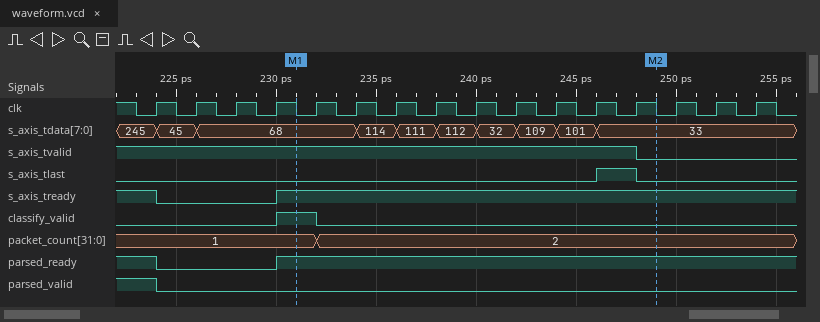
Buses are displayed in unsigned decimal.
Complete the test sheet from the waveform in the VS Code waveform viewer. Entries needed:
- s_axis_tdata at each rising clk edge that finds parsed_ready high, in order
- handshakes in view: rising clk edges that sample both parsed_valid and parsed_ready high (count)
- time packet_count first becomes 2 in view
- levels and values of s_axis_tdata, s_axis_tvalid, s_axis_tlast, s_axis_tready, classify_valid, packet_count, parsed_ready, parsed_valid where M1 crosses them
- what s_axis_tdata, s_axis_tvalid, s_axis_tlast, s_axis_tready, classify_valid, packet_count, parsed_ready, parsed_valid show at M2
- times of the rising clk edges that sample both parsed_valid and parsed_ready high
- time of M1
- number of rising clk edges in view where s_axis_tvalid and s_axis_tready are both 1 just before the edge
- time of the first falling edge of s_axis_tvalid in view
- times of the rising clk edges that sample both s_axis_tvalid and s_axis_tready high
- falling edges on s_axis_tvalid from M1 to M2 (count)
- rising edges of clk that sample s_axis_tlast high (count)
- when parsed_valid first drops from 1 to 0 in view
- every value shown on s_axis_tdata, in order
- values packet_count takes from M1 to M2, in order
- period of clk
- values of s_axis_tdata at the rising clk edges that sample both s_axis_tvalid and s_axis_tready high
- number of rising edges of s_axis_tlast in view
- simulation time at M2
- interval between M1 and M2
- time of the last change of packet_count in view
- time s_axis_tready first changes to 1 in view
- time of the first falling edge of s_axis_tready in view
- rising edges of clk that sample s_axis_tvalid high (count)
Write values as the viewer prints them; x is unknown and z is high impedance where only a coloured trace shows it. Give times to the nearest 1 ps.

245, 68, 68, 114, 111, 112, 32, 109, 101, 33, 33, 33, 33
1
232 ps
s_axis_tdata=68, s_axis_tvalid=1, s_axis_tlast=0, s_axis_tready=1, classify_valid=1, packet_count=1, parsed_ready=1, parsed_valid=0
s_axis_tdata=33, s_axis_tvalid=0, s_axis_tlast=0, s_axis_tready=1, classify_valid=0, packet_count=2, parsed_ready=1, parsed_valid=0
224 ps
231 ps
10
248 ps
224 ps, 232 ps, 234 ps, 236 ps, 238 ps, 240 ps, 242 ps, 244 ps, 246 ps, 248 ps
1
1
224 ps
245, 45, 68, 114, 111, 112, 32, 109, 101, 33
1, 2
2 ps
245, 68, 68, 114, 111, 112, 32, 109, 101, 33
1
249 ps
18 ps
232 ps
230 ps
224 ps
13
